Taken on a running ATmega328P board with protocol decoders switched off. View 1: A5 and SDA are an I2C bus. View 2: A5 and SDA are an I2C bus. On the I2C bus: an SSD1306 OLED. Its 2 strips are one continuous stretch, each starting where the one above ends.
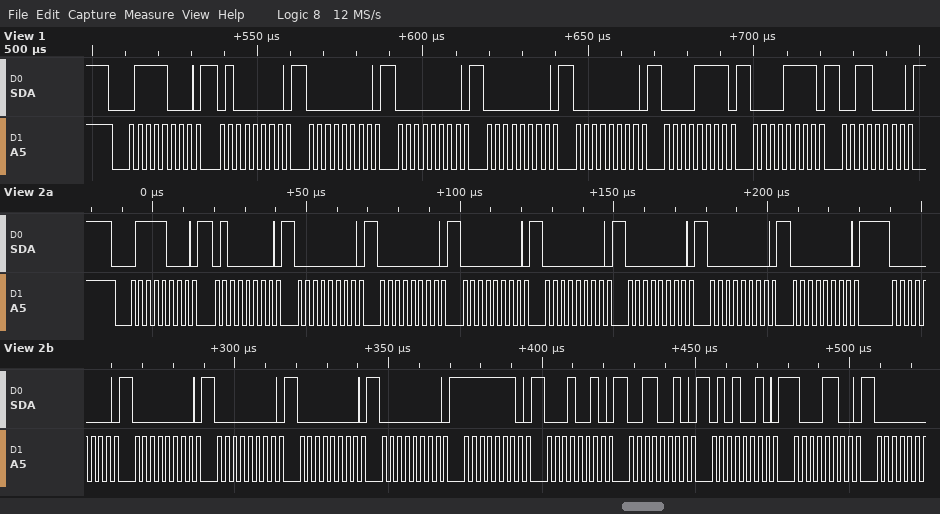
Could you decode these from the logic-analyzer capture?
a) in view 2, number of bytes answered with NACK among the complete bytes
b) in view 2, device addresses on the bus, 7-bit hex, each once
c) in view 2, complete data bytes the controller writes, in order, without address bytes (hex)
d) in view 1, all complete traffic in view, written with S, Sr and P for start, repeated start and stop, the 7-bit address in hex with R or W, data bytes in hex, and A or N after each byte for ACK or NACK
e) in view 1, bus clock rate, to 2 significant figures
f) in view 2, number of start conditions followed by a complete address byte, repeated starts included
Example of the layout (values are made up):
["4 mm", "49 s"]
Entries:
["0", "0x3C", "40 00 00 00 00 00 00 00 00 00 00 00 00 FE 12 32 52 8C", "S 3CW A 40 A 00 A 00 A 00 A 00 A 0F A 0F A 30 A", "400 kHz", "1"]
